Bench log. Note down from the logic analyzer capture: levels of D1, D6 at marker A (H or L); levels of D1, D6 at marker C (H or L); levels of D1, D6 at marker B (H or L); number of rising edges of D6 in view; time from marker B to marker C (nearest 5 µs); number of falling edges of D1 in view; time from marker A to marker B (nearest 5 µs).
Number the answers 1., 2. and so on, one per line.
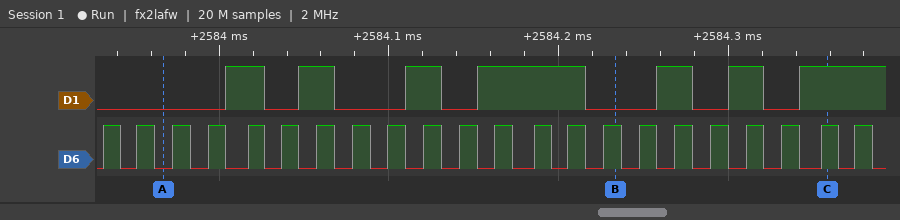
1. D1=L, D6=L
2. D1=H, D6=H
3. D1=L, D6=H
4. 22
5. 125 µs
6. 6
7. 265 µs
